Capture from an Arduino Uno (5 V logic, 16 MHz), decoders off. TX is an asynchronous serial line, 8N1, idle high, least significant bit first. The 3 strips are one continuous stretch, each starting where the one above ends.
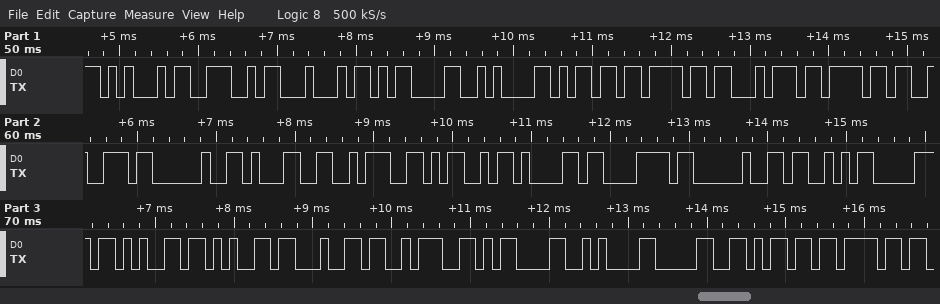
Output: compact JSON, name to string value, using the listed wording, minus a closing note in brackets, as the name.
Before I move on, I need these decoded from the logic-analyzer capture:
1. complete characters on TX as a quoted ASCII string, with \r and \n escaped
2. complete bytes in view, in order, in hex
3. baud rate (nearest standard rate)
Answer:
{"complete characters on TX as a quoted ASCII string, with \\r and \\n escaped": "\"END\\r\\nmotor 1:Max Speed:\\r\\n0mo\"", "complete bytes in view, in order, in hex": "0x45 0x4E 0x44 0x0D 0x0A 0x6D 0x6F 0x74 0x6F 0x72 0x20 0x31 0x3A 0x4D 0x61 0x78 0x20 0x53 0x70 0x65 0x65 0x64 0x3A 0x0D 0x0A 0x30 0x6D 0x6F", "baud rate": "9600 baud"}
